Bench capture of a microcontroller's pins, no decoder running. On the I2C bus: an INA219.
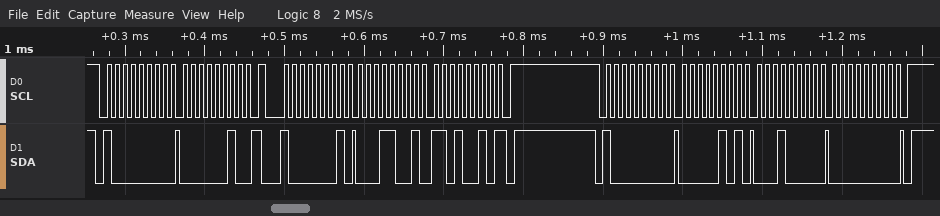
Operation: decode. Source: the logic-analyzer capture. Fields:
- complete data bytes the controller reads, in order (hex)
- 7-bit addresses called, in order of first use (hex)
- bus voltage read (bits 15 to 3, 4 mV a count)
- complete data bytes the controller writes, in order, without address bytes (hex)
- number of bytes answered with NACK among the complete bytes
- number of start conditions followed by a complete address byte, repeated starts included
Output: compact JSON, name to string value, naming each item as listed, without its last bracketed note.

{"complete data bytes the controller reads, in order": "19 D2", "7-bit addresses called, in order of first use": "0x40", "bus voltage read": "3.304 V", "complete data bytes the controller writes, in order, without address bytes": "02 05 10 00", "number of bytes answered with NACK among the complete bytes": "1", "number of start conditions followed by a complete address byte, repeated starts included": "3"}
